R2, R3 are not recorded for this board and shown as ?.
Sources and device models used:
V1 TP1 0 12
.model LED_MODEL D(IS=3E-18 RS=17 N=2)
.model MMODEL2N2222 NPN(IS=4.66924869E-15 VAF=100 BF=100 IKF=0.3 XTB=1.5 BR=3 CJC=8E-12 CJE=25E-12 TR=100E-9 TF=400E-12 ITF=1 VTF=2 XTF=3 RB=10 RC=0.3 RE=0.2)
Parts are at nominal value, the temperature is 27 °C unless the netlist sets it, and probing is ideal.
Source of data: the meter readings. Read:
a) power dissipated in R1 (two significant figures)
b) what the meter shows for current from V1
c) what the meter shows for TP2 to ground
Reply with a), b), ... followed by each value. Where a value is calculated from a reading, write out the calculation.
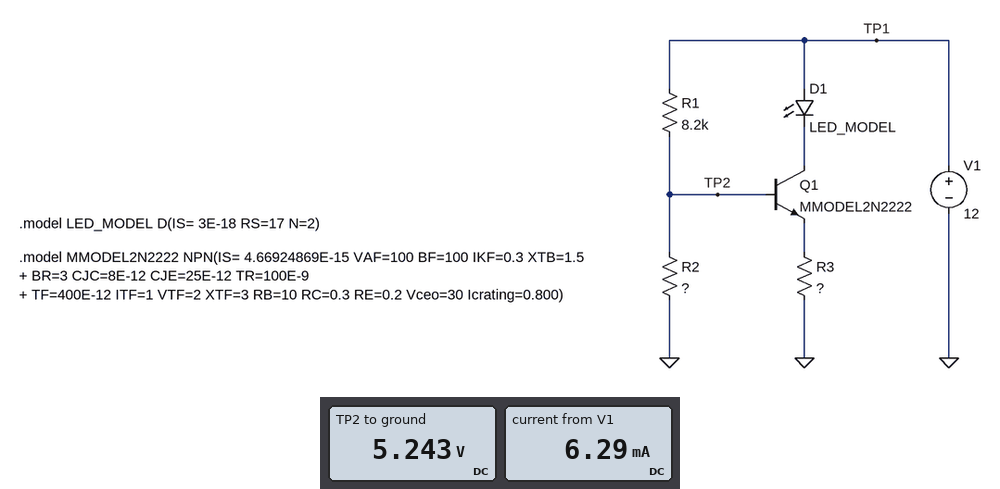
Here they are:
a) (12 V - 5.243 V)^2 / 8.2 kΩ = 5.6 mW
b) 6.29 mA
c) 5.243 V
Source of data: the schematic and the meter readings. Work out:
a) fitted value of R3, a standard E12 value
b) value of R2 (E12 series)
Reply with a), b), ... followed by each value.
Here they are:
a) 820 Ω
b) 6.8 kΩ
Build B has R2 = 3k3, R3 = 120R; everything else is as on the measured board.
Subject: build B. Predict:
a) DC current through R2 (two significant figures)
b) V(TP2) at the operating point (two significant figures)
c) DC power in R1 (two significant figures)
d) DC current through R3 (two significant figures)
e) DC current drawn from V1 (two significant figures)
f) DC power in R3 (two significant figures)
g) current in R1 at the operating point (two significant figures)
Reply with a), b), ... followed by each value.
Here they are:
a) 910 µA
b) 3.0 V
c) 9.9 mW
d) 19 mA
e) 20 mA
f) 42 mW
g) 1.1 mA
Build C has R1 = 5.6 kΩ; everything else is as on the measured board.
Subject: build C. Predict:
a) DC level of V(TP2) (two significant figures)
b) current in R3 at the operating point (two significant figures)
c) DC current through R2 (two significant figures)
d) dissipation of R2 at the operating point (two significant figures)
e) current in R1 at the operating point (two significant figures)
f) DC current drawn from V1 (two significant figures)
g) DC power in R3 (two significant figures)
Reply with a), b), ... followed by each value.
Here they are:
a) 6.4 V
b) 6.9 mA
c) 940 µA
d) 6.0 mW
e) 1.0 mA
f) 7.8 mA
g) 39 mW
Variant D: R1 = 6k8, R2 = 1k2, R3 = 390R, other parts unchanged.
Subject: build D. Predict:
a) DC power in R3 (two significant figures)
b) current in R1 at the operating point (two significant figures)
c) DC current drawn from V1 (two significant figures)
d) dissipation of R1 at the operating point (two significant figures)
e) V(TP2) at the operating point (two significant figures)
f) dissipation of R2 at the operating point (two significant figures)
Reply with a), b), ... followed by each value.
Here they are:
a) 3.0 mW
b) 1.5 mA
c) 4.2 mA
d) 15 mW
e) 1.8 V
f) 2.6 mW
